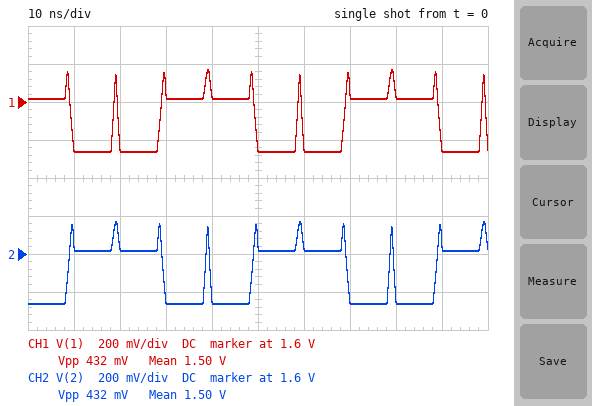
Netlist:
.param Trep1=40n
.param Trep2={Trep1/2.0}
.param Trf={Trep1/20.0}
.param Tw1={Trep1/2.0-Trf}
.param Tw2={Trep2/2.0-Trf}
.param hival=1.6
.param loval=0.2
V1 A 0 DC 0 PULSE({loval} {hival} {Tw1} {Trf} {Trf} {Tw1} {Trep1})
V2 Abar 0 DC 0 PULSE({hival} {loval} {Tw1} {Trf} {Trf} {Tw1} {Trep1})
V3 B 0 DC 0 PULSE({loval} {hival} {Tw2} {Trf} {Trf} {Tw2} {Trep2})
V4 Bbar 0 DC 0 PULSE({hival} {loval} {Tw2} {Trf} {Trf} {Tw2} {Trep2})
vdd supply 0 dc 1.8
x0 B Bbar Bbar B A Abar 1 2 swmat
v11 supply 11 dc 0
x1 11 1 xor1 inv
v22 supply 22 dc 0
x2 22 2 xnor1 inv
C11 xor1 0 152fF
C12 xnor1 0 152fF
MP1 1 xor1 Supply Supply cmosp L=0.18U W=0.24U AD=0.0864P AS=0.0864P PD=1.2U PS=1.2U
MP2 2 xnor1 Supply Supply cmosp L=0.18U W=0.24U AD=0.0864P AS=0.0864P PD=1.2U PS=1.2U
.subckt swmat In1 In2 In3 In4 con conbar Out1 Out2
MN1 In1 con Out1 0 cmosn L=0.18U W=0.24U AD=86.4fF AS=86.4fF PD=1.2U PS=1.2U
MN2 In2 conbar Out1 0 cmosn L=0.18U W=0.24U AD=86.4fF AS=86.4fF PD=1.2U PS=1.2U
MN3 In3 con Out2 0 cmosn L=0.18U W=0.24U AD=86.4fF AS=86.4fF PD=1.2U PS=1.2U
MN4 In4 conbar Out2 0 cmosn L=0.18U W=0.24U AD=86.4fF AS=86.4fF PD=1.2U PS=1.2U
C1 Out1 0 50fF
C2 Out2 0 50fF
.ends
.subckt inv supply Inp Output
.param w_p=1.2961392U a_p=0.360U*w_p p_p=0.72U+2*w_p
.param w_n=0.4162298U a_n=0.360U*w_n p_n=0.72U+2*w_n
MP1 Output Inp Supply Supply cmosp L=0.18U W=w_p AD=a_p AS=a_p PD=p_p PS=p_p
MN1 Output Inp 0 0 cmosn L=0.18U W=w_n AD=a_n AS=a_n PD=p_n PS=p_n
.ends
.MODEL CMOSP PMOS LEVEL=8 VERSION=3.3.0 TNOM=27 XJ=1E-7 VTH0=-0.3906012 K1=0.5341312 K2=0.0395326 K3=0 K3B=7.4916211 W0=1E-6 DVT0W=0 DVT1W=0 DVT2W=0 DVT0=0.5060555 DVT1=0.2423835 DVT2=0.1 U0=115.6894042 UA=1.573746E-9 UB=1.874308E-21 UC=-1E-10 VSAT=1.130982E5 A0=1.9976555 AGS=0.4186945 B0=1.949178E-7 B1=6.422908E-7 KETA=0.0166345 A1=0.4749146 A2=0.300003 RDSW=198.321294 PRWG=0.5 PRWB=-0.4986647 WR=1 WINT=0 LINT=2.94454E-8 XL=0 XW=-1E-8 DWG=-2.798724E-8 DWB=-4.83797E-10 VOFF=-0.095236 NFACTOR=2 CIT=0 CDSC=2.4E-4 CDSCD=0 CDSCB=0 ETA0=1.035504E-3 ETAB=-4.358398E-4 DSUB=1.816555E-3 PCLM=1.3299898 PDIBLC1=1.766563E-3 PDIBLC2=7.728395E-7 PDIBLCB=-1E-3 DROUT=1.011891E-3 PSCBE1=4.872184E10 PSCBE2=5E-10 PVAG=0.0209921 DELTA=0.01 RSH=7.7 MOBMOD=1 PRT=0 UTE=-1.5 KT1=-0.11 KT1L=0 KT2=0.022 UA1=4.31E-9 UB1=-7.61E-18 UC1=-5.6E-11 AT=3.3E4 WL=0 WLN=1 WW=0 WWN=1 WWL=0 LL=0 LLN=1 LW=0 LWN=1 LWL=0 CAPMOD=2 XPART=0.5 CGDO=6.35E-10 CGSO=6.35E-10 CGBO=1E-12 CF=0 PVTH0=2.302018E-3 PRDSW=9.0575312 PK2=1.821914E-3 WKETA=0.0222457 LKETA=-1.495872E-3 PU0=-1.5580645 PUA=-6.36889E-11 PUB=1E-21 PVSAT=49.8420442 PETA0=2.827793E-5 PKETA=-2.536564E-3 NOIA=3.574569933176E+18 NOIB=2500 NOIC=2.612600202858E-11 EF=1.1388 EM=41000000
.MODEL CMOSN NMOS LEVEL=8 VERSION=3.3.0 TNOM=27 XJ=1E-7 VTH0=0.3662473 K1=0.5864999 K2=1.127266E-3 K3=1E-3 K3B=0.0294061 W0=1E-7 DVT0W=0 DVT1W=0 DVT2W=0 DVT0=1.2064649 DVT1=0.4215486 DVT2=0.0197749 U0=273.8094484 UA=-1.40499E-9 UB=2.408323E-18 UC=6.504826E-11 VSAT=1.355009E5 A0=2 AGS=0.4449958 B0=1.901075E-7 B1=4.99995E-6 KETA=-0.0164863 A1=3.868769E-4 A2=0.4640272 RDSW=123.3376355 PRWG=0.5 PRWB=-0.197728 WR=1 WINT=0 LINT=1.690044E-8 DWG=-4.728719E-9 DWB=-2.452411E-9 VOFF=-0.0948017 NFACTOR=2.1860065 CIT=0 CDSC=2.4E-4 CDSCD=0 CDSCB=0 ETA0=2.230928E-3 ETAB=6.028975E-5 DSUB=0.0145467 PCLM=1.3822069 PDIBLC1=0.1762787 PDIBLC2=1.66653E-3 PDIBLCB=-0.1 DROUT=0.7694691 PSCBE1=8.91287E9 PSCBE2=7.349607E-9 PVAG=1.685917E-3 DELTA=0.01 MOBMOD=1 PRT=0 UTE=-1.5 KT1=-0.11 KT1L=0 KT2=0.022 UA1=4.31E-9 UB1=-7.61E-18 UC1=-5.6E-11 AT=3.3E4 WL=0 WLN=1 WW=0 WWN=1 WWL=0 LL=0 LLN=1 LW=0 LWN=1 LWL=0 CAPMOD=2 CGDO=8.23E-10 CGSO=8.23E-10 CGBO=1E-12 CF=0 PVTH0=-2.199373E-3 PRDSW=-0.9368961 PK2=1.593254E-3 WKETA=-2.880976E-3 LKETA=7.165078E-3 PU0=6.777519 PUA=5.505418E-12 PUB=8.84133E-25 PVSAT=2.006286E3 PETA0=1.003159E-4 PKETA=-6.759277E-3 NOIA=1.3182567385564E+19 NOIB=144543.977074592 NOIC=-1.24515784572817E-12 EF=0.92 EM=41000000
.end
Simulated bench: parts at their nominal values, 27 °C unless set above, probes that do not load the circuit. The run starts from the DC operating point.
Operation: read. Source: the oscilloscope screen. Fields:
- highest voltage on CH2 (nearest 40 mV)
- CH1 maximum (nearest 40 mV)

1.76 V
1.76 V
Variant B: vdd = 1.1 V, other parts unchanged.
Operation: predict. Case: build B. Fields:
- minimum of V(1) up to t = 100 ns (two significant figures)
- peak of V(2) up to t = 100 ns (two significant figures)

760 mV
1.1 V
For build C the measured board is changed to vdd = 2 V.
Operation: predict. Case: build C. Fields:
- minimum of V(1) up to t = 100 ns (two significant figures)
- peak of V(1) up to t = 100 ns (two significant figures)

1.5 V
1.9 V
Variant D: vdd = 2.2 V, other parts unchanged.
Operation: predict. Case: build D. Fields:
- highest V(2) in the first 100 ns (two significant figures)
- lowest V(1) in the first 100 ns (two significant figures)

2.1 V
1.7 V
